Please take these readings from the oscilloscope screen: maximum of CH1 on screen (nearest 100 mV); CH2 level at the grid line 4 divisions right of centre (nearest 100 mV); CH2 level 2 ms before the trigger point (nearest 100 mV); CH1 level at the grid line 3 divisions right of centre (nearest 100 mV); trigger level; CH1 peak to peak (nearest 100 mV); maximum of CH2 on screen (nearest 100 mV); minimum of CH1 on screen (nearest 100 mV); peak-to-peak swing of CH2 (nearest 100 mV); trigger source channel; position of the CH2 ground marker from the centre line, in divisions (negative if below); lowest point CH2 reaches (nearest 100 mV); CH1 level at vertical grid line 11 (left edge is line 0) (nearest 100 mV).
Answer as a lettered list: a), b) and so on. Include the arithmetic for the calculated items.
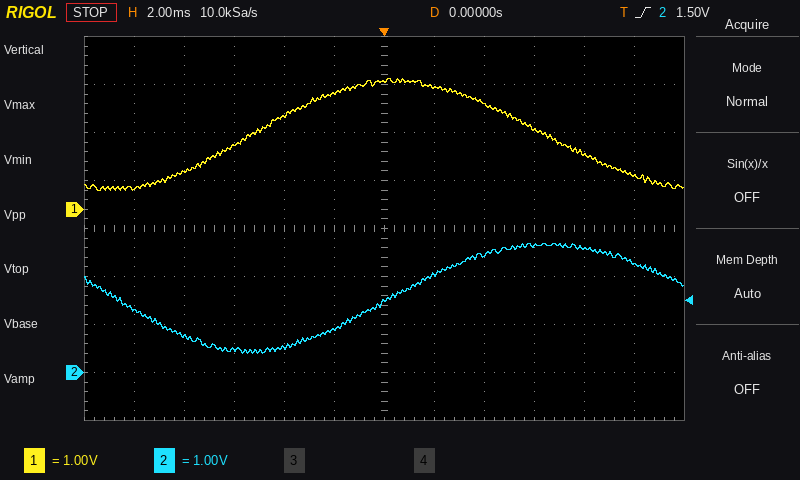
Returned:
a) 2.7 V
b) 2.6 V
c) 900 mV
d) 1.7 V
e) 1.50 V
f) 2.7 V − (400 mV) = 2.3 V
g) 2.7 V
h) 400 mV
i) 2.7 V − (400 mV) = 2.3 V
j) CH2
k) -3.0 div
l) 400 mV
m) 700 mV
